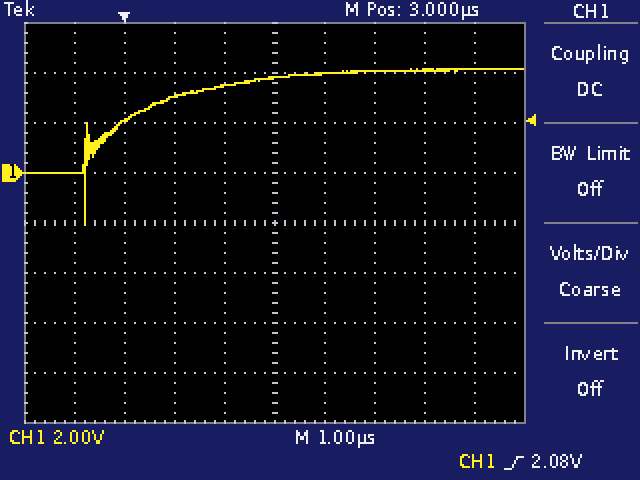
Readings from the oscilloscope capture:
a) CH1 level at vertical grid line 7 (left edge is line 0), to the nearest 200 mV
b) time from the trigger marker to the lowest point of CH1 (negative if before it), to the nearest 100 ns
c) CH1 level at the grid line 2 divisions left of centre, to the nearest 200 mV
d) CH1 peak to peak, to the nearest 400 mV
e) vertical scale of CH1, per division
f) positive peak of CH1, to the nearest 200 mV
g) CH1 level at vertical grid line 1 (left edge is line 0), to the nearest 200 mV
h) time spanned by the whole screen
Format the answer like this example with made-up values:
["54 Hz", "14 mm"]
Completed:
["4.0 V", "-800 ns", "3.0 V", "6.4 V", "2 V", "4.2 V", "0.0 V", "10 µs"]
